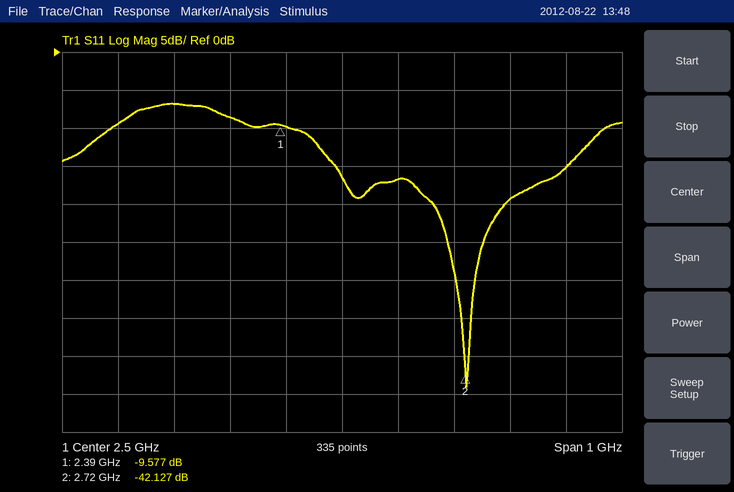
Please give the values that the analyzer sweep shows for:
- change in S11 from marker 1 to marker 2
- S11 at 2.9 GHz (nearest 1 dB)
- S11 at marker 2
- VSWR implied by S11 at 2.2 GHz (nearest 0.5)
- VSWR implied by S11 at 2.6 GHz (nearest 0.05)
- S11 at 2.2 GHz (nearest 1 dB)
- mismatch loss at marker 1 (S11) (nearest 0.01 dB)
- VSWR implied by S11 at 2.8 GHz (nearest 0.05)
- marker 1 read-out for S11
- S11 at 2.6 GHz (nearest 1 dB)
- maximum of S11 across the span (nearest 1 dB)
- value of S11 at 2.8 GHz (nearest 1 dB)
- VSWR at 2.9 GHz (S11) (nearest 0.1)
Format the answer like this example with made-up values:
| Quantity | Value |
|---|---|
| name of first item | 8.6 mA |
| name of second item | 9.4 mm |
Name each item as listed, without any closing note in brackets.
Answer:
| Quantity | Value |
|---|---|
| change in S11 from marker 1 to marker 2 | -32.550 dB |
| S11 at 2.9 GHz | -15 dB |
| S11 at marker 2 | -42.127 dB |
| VSWR implied by S11 at 2.2 GHz | 2.5 |
| VSWR implied by S11 at 2.6 GHz | 1.35 |
| S11 at 2.2 GHz | -7 dB |
| mismatch loss at marker 1 (S11) | 0.51 dB |
| VSWR implied by S11 at 2.8 GHz | 1.25 |
| marker 1 read-out for S11 | -9.577 dB |
| S11 at 2.6 GHz | -17 dB |
| maximum of S11 across the span | -7 dB |
| value of S11 at 2.8 GHz | -19 dB |
| VSWR at 2.9 GHz (S11) | 1.4 |
